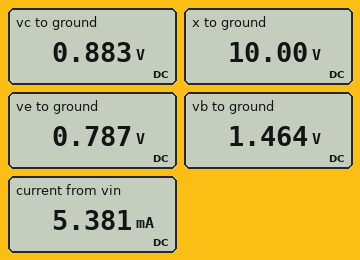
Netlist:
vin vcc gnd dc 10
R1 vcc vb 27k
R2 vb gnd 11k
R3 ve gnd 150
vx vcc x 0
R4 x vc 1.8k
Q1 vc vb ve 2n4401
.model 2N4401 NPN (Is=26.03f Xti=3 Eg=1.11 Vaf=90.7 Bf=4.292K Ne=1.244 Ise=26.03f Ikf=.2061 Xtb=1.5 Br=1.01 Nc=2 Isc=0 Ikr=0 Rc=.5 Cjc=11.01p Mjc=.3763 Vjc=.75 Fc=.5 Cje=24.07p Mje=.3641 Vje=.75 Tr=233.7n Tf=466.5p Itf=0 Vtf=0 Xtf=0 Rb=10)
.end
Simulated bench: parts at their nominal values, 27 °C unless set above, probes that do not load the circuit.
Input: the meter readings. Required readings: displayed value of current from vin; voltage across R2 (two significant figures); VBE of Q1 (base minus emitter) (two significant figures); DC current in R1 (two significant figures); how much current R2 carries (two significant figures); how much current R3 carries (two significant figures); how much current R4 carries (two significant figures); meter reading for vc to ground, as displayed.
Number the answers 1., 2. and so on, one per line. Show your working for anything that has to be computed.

1. 5.381 mA
2. 1.464 V = 1.5 V
3. 1.464 V - 787 mV = 680 mV
4. (10 V - 1.464 V) / 27 kΩ = 320 µA
5. (1.464 V) / 11 kΩ = 130 µA
6. (787 mV) / 150 Ω = 5.2 mA
7. (10 V - 883 mV) / 1.8 kΩ = 5.1 mA
8. 0.883 V
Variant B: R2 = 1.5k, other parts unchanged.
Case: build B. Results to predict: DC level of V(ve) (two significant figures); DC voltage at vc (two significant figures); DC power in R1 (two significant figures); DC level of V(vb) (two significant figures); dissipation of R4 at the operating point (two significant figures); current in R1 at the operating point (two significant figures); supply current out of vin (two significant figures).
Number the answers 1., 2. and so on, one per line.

1. 2.7 mV
2. 10 V
3. 3.3 mW
4. 530 mV
5. 550 nW
6. 350 µA
7. 370 µA
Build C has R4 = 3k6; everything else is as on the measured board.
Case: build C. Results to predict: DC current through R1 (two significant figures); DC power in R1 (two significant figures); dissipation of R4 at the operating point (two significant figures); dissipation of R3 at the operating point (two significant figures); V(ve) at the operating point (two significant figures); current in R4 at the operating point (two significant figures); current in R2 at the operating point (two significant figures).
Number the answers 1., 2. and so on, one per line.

1. 330 µA
2. 2.9 mW
3. 25 mW
4. 1.2 mW
5. 430 mV
6. 2.6 mA
7. 99 µA
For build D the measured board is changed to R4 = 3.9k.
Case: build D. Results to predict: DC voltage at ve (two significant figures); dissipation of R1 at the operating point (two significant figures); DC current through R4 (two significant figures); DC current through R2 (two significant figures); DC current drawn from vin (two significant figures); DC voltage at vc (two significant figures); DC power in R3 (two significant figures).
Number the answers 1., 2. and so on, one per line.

1. 400 mV
2. 3.0 mW
3. 2.4 mA
4. 97 µA
5. 2.8 mA
6. 470 mV
7. 1.1 mW
